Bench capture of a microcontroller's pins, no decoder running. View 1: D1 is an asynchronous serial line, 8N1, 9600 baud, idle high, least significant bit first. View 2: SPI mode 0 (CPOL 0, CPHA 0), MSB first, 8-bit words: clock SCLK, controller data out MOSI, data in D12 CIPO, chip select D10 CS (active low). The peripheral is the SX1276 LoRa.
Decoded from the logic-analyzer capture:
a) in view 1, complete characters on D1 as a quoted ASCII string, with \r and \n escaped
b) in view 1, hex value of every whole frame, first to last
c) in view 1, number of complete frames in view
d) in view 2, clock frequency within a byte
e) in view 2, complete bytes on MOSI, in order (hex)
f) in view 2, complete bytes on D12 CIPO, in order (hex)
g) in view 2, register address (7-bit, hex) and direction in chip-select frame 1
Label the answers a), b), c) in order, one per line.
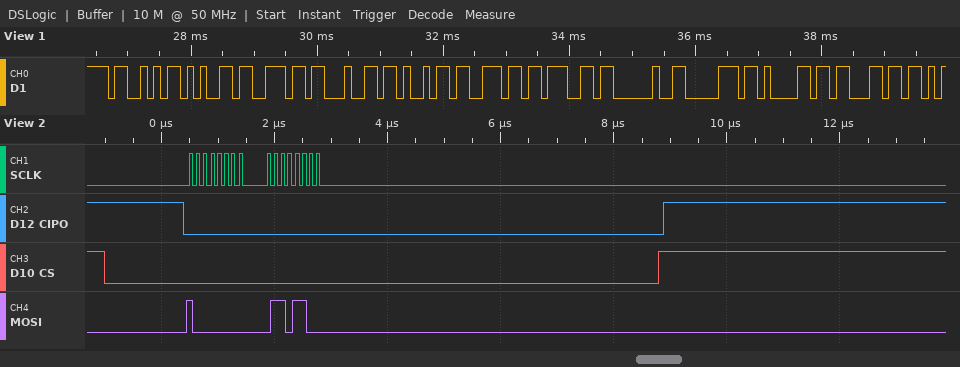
a) "Sending pac"
b) 0x53 0x65 0x6E 0x64 0x69 0x6E 0x67 0x20 0x70 0x61 0x63
c) 11
d) 8 MHz
e) 0x80 0x6C
f) 0x00 0x00
g) 0x00 write
